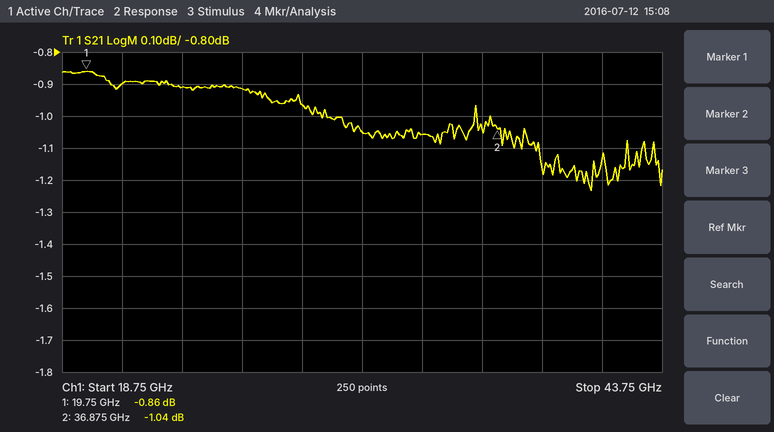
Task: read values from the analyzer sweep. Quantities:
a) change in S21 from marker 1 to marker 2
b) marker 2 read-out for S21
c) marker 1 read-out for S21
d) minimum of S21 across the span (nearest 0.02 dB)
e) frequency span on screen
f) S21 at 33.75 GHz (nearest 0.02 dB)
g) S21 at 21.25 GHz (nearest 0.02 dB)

-0.18 dB
-1.04 dB
-0.86 dB
-1.24 dB
25 GHz
-1.06 dB
-0.90 dB
